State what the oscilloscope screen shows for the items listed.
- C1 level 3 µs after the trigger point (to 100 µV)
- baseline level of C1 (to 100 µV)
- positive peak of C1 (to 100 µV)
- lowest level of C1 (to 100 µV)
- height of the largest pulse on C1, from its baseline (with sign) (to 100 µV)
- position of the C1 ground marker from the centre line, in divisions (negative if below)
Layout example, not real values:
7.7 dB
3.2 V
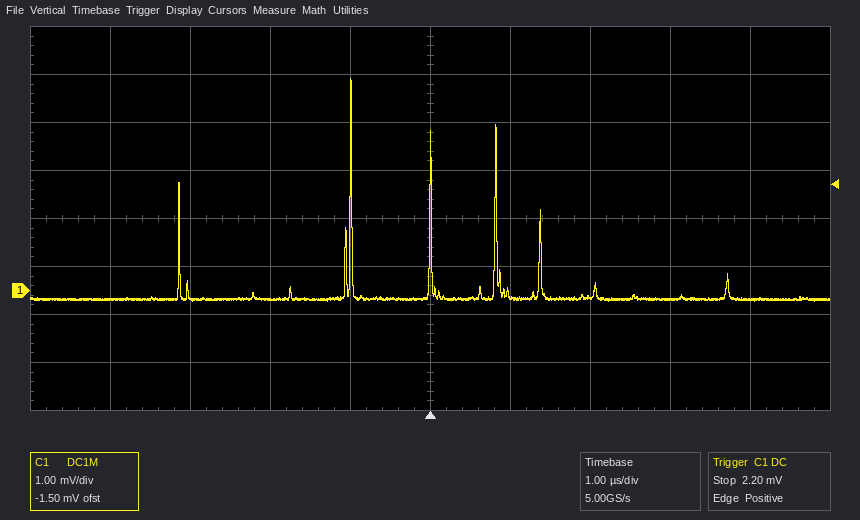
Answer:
-200 µV
-200 µV
4.4 mV
-200 µV
+4.6 mV
-1.5 div
